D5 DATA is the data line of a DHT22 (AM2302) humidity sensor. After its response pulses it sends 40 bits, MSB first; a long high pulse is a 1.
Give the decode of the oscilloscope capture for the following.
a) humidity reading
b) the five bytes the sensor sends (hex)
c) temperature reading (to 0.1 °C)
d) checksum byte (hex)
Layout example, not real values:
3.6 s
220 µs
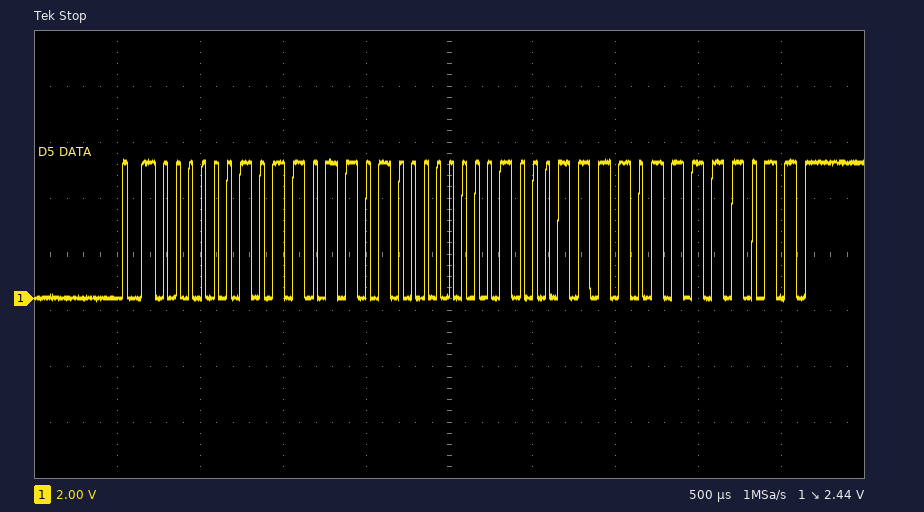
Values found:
73.0 %
02 DA 01 1E FB
28.6 °C
0xFB
